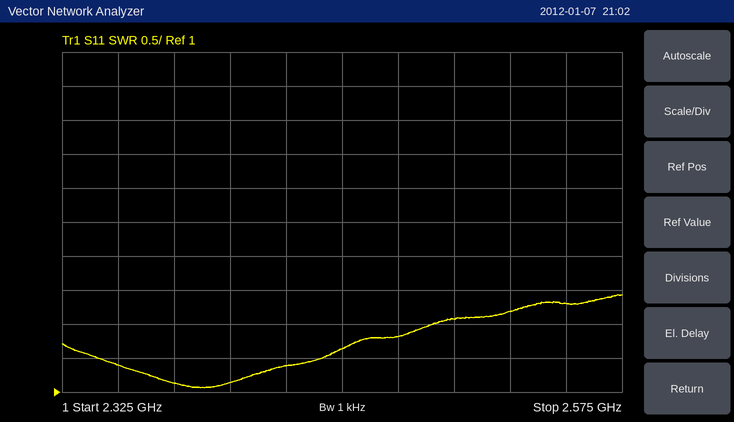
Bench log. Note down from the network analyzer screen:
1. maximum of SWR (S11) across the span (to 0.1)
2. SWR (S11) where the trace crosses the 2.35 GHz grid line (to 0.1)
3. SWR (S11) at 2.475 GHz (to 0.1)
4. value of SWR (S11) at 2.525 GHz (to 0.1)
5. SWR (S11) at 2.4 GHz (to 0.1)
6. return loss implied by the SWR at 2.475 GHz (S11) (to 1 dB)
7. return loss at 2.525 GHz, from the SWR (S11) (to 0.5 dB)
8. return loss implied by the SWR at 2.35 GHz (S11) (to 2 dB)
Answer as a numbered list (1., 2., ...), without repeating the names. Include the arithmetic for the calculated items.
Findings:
1. 2.4
2. 1.4
3. 1.8
4. 2.2
5. 1.1
6. −20 log10((1.8 − 1)/(1.8 + 1)) ≈ 11 dB
7. −20 log10((2.2 − 1)/(2.2 + 1)) ≈ 8.5 dB
8. −20 log10((1.4 − 1)/(1.4 + 1)) ≈ 16 dB
